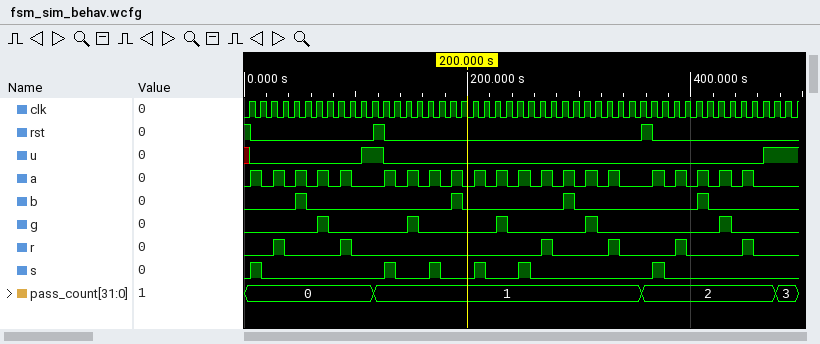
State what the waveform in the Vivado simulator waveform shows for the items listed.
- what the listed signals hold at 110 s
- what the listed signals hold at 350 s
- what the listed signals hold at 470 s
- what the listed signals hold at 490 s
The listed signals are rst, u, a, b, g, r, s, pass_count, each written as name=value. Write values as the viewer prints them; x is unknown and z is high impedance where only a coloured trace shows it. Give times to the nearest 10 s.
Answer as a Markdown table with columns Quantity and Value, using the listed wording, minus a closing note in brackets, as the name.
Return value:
| Quantity | Value |
|---|---|
| what the listed signals hold at 110 s | rst=0, u=1, a=0, b=0, g=0, r=0, s=0, pass_count=0 |
| what the listed signals hold at 350 s | rst=0, u=0, a=0, b=0, g=0, r=0, s=0, pass_count=1 |
| what the listed signals hold at 470 s | rst=0, u=1, a=0, b=0, g=0, r=0, s=0, pass_count=2 |
| what the listed signals hold at 490 s | rst=0, u=1, a=0, b=0, g=0, r=0, s=0, pass_count=3 |
